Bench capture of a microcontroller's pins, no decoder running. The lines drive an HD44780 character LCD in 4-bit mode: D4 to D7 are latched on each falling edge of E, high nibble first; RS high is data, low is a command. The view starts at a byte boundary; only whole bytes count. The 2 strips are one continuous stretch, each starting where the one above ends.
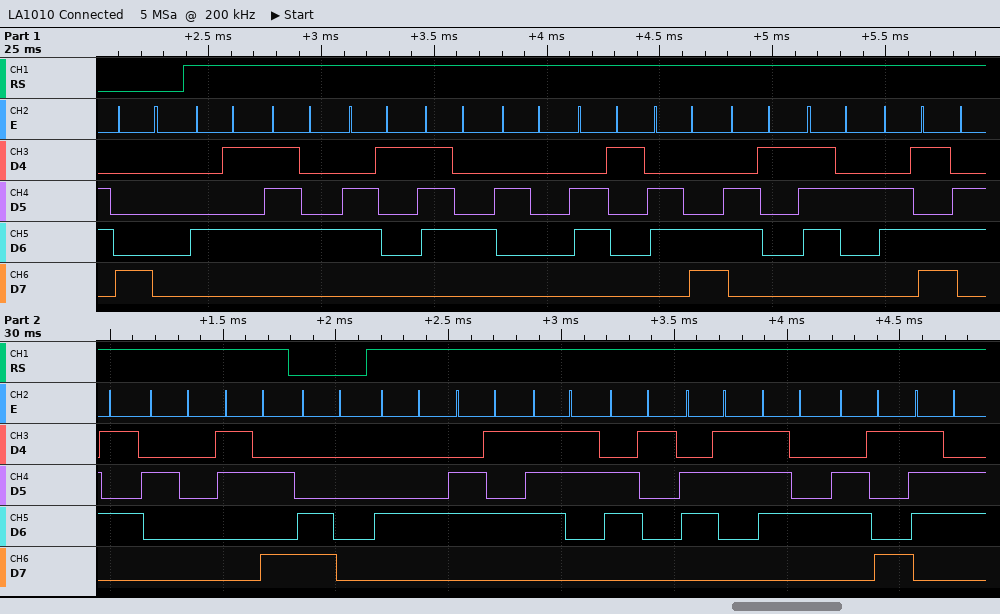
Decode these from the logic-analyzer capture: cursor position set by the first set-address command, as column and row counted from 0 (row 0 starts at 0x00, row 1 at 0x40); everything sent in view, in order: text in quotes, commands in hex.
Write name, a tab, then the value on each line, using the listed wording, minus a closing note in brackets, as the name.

cursor position set by the first set-address command, as column and row counted from 0	column 0, row 0
everything sent in view, in order: text in quotes, commands in hex	0x80 "Etat alarme :" 0xC0 "Desactiv"
